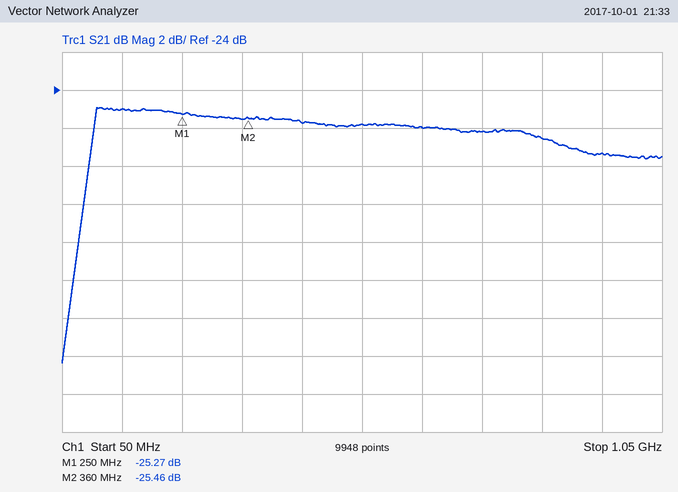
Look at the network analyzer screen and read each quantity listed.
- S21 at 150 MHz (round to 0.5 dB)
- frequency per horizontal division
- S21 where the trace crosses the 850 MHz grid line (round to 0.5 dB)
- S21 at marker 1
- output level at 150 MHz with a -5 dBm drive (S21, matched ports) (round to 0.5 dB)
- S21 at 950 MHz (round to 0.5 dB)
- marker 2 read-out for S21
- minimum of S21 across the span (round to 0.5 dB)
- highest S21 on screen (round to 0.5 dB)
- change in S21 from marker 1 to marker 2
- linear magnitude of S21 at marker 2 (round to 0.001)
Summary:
-25.0 dB
100 MHz
-26.5 dB
-25.27 dB
-30.0 dBm
-27.5 dB
-25.46 dB
-38.5 dB
-25.0 dB
-0.19 dB
0.053
